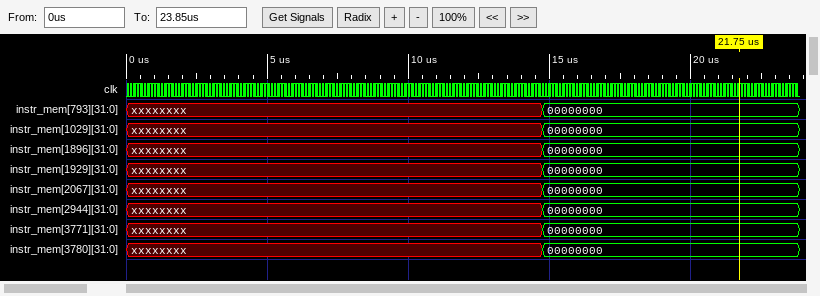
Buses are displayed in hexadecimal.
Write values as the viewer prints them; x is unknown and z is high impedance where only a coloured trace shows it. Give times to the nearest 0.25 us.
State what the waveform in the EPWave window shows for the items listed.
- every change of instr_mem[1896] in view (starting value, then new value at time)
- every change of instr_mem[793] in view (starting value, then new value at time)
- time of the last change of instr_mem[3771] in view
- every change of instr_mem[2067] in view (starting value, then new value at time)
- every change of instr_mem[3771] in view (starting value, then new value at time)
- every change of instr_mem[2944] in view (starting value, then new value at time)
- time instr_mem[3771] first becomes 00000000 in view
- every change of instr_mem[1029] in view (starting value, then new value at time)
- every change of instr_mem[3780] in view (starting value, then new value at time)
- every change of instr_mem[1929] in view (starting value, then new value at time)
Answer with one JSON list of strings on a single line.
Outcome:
["xxxxxxxx, 00000000 at 14.75 us", "xxxxxxxx, 00000000 at 14.75 us", "14.75 us", "xxxxxxxx, 00000000 at 14.75 us", "xxxxxxxx, 00000000 at 14.75 us", "xxxxxxxx, 00000000 at 14.75 us", "14.75 us", "xxxxxxxx, 00000000 at 14.75 us", "xxxxxxxx, 00000000 at 14.75 us", "xxxxxxxx, 00000000 at 14.75 us"]
